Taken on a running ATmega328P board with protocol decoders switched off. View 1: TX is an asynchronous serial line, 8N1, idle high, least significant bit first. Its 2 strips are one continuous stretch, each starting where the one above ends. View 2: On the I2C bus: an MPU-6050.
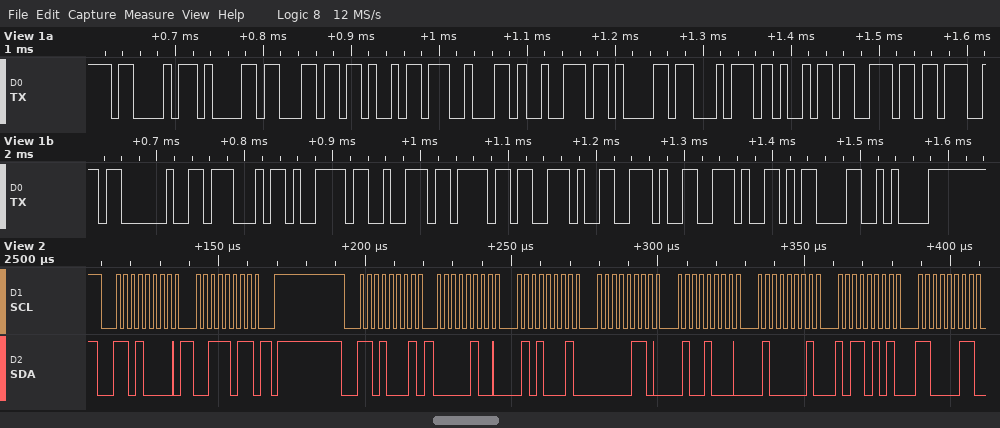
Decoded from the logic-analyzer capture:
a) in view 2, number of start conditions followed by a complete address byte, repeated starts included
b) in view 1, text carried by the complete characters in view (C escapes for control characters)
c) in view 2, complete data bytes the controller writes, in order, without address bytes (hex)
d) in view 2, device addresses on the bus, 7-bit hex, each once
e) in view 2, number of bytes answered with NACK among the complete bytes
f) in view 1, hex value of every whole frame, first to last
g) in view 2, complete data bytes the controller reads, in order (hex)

2
"Calibrating Gyro...\r\n"
3B
0x68
0
0x43 0x61 0x6C 0x69 0x62 0x72 0x61 0x74 0x69 0x6E 0x67 0x20 0x47 0x79 0x72 0x6F 0x2E 0x2E 0x2E 0x0D 0x0A
04 51 06 48 41 B5 C3
